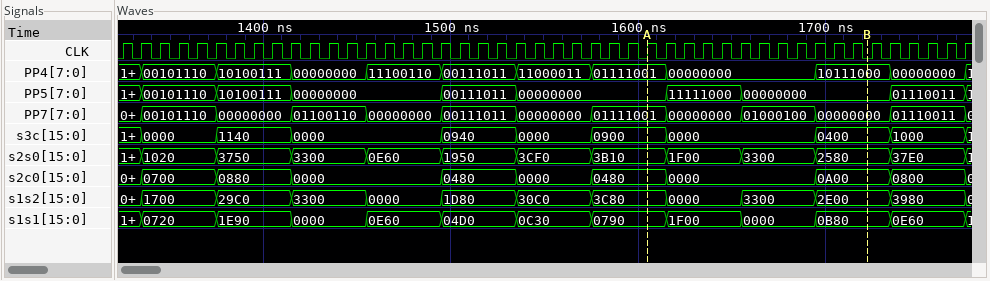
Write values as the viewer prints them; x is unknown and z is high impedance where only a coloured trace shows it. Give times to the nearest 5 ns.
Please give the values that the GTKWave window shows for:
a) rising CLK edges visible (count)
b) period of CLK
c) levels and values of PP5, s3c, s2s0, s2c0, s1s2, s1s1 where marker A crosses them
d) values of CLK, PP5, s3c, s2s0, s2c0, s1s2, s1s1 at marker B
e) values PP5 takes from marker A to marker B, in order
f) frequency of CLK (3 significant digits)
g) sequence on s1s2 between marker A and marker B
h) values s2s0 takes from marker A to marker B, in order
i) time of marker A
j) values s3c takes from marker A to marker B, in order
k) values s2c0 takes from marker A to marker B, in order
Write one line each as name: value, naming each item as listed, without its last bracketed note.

rising CLK edges visible: 46
period of CLK: 10 ns
levels and values of PP5, s3c, s2s0, s2c0, s1s2, s1s1 where marker A crosses them: PP5=00000000, s3c=0900, s2s0=3B10, s2c0=0480, s1s2=3C80, s1s1=0790
values of CLK, PP5, s3c, s2s0, s2c0, s1s2, s1s1 at marker B: CLK=0, PP5=00000000, s3c=0400, s2s0=2580, s2c0=0A00, s1s2=2E00, s1s1=0B80
values PP5 takes from marker A to marker B, in order: 00000000, 11111000, 00000000
frequency of CLK: 100 MHz
sequence on s1s2 between marker A and marker B: 3C80, 0000, 3300, 2E00
values s2s0 takes from marker A to marker B, in order: 3B10, 1F00, 3300, 2580
time of marker A: 1605 ns
values s3c takes from marker A to marker B, in order: 0900, 0000, 0400
values s2c0 takes from marker A to marker B, in order: 0480, 0000, 0A00
